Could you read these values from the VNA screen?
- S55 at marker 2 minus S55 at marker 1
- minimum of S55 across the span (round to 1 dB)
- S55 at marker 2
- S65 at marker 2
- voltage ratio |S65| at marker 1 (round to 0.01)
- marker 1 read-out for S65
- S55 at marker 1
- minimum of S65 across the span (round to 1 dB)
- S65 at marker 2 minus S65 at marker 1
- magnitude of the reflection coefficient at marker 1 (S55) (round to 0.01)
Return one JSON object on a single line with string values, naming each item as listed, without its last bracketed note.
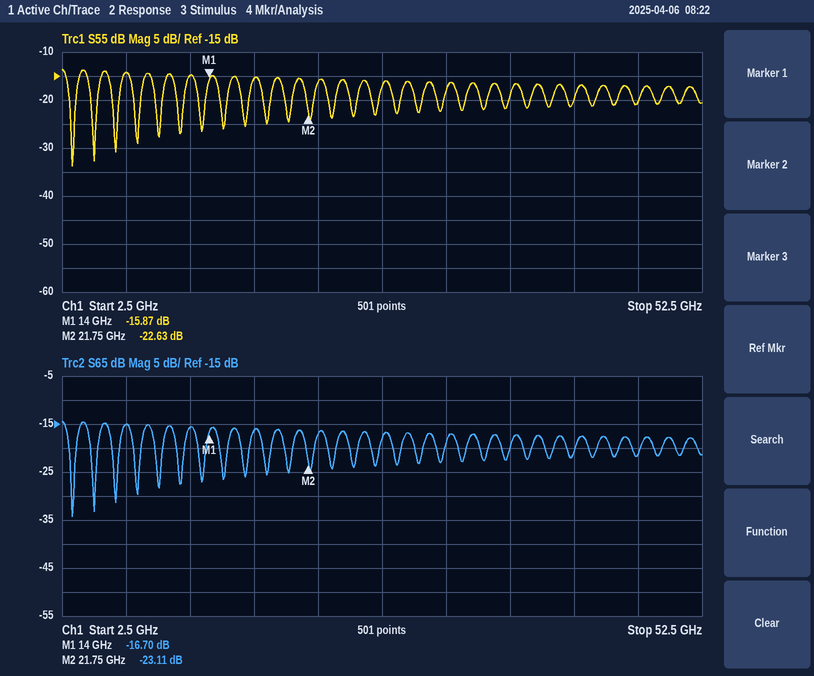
{"S55 at marker 2 minus S55 at marker 1": "-6.76 dB", "minimum of S55 across the span": "-34 dB", "S55 at marker 2": "-22.63 dB", "S65 at marker 2": "-23.11 dB", "voltage ratio |S65| at marker 1": "0.15", "marker 1 read-out for S65": "-16.70 dB", "S55 at marker 1": "-15.87 dB", "minimum of S65 across the span": "-34 dB", "S65 at marker 2 minus S65 at marker 1": "-6.41 dB", "magnitude of the reflection coefficient at marker 1 (S55)": "0.16"}
